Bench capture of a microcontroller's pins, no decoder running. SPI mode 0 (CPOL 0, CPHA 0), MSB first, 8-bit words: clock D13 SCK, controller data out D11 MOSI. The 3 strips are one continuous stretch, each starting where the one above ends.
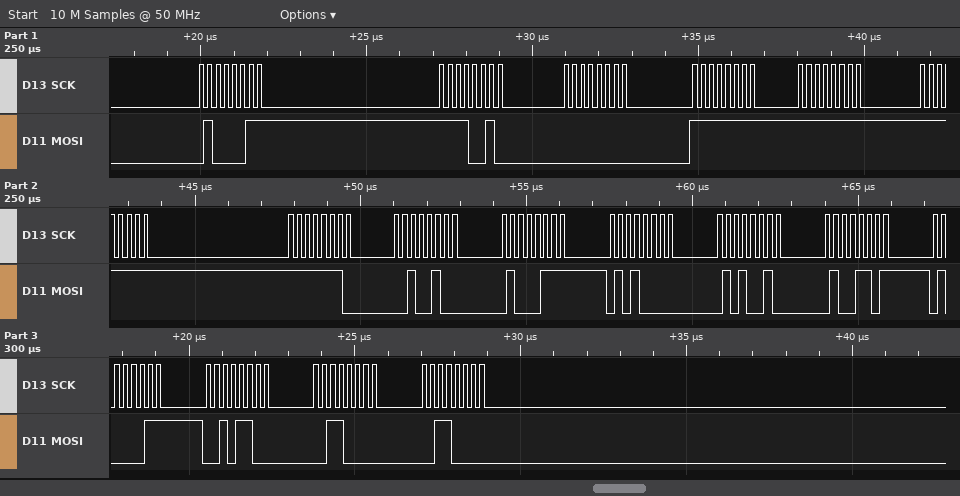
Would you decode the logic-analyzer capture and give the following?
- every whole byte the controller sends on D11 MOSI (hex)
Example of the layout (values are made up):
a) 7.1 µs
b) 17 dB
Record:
a) 0x43 0xF2 0x00 0xFF 0xFF 0xFF 0xFE 0x24 0x47 0x50 0x52 0x4D 0x43 0x2C 0x30 0x30
